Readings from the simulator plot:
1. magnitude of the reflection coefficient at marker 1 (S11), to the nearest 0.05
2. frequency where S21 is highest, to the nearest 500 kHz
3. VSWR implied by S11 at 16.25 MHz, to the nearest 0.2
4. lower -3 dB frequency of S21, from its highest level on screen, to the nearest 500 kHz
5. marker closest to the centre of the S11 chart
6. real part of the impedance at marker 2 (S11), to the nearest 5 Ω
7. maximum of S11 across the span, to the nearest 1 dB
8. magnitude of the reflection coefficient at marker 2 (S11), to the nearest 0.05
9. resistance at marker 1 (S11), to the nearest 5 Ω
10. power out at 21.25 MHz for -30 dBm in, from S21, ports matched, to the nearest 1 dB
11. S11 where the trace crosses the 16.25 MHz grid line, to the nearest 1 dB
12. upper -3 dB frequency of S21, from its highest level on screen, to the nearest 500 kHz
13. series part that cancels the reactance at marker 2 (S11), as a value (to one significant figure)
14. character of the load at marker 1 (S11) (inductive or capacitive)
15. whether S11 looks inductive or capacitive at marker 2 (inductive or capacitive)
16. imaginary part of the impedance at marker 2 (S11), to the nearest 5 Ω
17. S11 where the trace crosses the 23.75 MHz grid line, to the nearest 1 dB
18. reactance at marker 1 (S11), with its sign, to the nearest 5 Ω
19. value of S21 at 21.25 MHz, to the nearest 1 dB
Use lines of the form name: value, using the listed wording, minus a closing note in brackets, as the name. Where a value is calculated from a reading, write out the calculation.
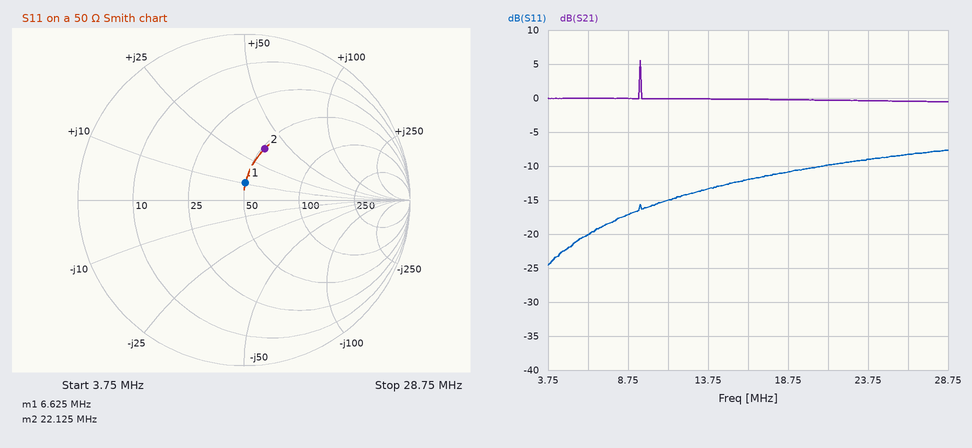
magnitude of the reflection coefficient at marker 1 (S11), to the nearest 0.05: 0.10
frequency where S21 is highest, to the nearest 500 kHz: 9.5 MHz
VSWR implied by S11 at 16.25 MHz, to the nearest 0.2: |Γ| = 10^(-12/20) = 0.2512; VSWR = (1 + 0.2512)/(1 − 0.2512) ≈ 1.67, so 1.6 to the nearest 0.2
lower -3 dB frequency of S21, from its highest level on screen, to the nearest 500 kHz: 9.5 MHz
marker closest to the centre of the S11 chart: marker 1
real part of the impedance at marker 2 (S11), to the nearest 5 Ω: 50 Ω
maximum of S11 across the span, to the nearest 1 dB: -8 dB
magnitude of the reflection coefficient at marker 2 (S11), to the nearest 0.05: 0.35
resistance at marker 1 (S11), to the nearest 5 Ω: 50 Ω
power out at 21.25 MHz for -30 dBm in, from S21, ports matched, to the nearest 1 dB: -30 dBm + (0 dB) = -30 dBm
S11 where the trace crosses the 16.25 MHz grid line, to the nearest 1 dB: -12 dB
upper -3 dB frequency of S21, from its highest level on screen, to the nearest 500 kHz: 9.5 MHz
series part that cancels the reactance at marker 2 (S11), as a value: C = 1/(2π × 22.125 MHz × 35 Ω) ≈ 206 pF, so 200 pF to one significant figure
character of the load at marker 1 (S11): inductive
whether S11 looks inductive or capacitive at marker 2: inductive
imaginary part of the impedance at marker 2 (S11), to the nearest 5 Ω: +35 Ω
S11 where the trace crosses the 23.75 MHz grid line, to the nearest 1 dB: -9 dB
reactance at marker 1 (S11), with its sign, to the nearest 5 Ω: +10 Ω
value of S21 at 21.25 MHz, to the nearest 1 dB: 0 dB
